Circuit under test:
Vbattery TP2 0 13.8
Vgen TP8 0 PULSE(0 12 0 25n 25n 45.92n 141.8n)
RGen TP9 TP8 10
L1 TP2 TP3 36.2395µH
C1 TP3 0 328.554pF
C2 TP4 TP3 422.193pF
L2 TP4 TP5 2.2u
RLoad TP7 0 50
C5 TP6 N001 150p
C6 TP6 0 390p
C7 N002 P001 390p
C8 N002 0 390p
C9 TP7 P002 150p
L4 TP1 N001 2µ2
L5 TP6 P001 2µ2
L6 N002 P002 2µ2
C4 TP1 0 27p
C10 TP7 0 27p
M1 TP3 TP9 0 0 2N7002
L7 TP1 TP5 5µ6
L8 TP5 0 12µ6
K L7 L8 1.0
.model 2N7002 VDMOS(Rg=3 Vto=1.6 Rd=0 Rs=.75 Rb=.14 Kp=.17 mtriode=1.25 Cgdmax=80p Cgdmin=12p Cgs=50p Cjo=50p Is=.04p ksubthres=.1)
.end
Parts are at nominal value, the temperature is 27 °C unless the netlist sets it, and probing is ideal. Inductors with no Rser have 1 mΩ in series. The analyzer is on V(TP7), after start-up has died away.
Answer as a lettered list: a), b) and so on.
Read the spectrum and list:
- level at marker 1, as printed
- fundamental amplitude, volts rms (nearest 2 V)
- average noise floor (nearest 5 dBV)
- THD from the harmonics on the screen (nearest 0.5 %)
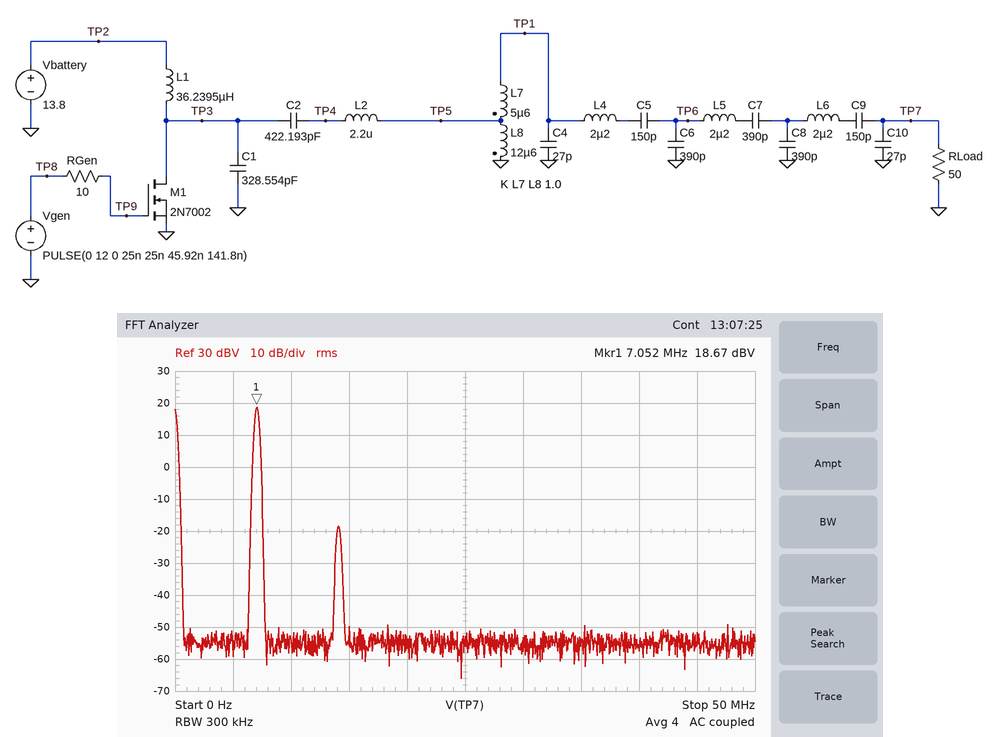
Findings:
a) 18.67 dBV
b) 8 V
c) -55 dBV
d) 1.5 %
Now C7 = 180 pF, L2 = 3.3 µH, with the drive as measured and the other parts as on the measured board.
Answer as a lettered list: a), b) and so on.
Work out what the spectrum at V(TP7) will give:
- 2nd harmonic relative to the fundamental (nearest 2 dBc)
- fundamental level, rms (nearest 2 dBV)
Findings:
a) -24 dBc
b) 4 dBV
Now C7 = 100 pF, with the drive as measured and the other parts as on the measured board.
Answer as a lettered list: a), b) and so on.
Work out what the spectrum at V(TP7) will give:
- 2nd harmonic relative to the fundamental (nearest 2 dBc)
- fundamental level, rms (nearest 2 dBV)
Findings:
a) -14 dBc
b) 14 dBV
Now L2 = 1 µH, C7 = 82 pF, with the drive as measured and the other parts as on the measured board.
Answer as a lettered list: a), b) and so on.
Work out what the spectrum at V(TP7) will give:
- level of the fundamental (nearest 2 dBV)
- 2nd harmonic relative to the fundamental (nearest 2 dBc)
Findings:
a) 0 dBV
b) 8 dBc
